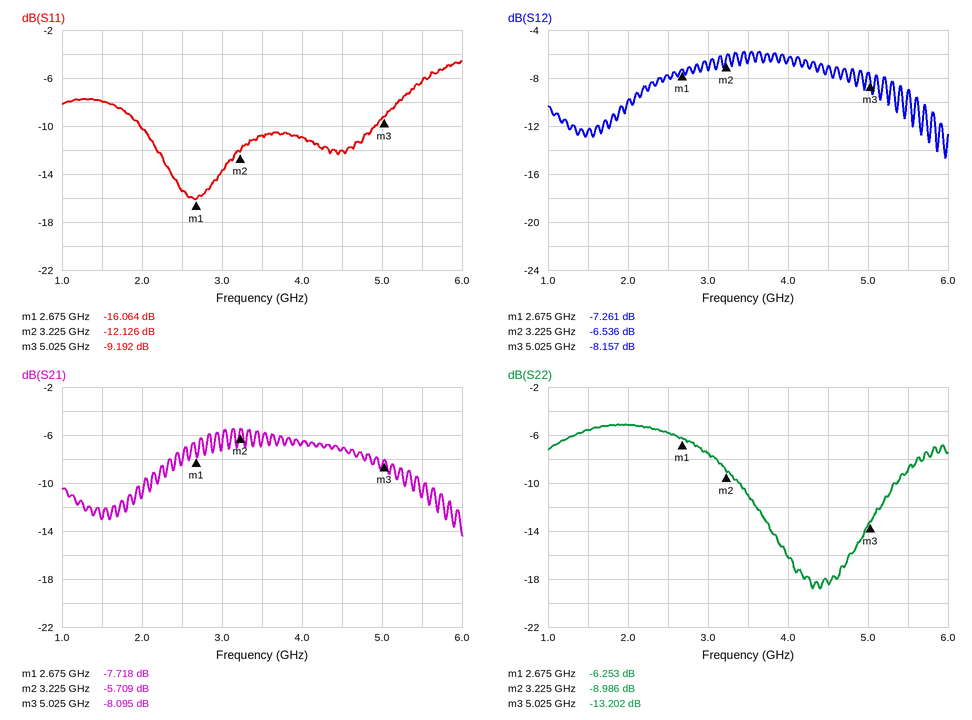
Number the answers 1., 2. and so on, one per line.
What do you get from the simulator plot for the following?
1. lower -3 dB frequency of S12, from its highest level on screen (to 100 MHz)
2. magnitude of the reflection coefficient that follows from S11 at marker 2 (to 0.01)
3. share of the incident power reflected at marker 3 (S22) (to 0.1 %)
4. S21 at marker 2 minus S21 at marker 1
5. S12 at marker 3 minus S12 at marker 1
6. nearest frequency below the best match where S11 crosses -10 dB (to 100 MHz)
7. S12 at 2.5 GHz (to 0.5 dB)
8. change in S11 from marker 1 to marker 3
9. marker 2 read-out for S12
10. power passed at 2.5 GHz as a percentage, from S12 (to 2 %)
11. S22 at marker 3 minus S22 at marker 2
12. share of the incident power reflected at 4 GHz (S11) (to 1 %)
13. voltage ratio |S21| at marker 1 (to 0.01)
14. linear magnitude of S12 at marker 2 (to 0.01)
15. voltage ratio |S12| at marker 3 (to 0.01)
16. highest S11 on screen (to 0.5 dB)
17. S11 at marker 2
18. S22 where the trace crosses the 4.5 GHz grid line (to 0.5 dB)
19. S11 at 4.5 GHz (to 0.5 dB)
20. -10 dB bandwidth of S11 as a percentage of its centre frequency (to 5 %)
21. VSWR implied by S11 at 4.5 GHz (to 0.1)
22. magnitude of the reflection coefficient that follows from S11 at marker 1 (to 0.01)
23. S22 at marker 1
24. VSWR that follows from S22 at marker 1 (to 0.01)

1. 2.3 GHz
2. 0.25
3. 4.8 %
4. 2.009 dB
5. -0.896 dB
6. 2.0 GHz
7. -8.0 dB
8. 6.872 dB
9. -6.536 dB
10. 16 %
11. -4.216 dB
12. 8 %
13. 0.41
14. 0.47
15. 0.39
16. -4.5 dB
17. -12.126 dB
18. -18.5 dB
19. -12.0 dB
20. 85 %
21. 1.7
22. 0.16
23. -6.253 dB
24. 2.90
